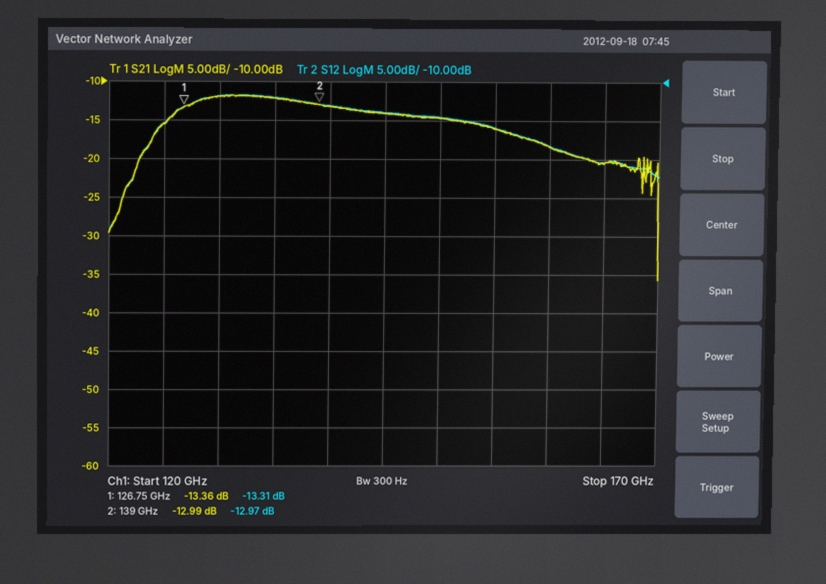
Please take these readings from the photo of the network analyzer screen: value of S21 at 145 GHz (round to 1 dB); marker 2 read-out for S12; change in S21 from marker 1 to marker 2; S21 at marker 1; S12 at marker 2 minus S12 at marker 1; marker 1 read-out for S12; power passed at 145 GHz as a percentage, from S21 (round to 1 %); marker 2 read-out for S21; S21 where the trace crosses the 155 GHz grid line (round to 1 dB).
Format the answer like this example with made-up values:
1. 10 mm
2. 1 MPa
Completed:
1. -14 dB
2. -12.97 dB
3. 0.37 dB
4. -13.36 dB
5. 0.34 dB
6. -13.31 dB
7. 4 %
8. -12.99 dB
9. -16 dB
